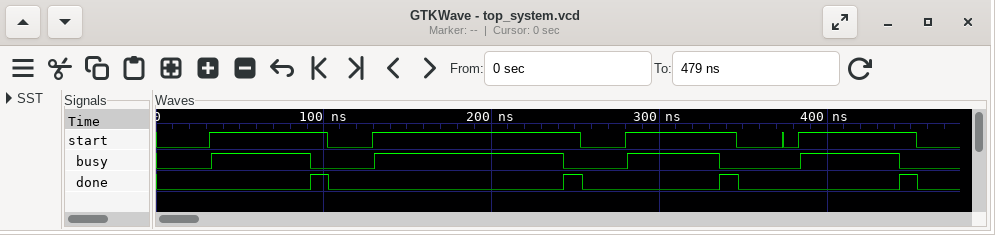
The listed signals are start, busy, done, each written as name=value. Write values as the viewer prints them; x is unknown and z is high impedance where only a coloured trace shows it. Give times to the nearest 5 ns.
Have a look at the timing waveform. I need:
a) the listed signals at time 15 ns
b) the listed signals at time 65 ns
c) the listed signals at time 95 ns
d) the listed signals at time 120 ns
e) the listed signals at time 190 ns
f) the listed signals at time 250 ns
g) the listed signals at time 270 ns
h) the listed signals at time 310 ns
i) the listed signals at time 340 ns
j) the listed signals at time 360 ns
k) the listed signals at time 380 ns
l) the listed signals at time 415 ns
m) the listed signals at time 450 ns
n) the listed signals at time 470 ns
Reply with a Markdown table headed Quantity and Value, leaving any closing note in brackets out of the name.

| Quantity | Value |
|---|---|
| the listed signals at time 15 ns | start=0, busy=0, done=0 |
| the listed signals at time 65 ns | start=1, busy=1, done=0 |
| the listed signals at time 95 ns | start=1, busy=0, done=1 |
| the listed signals at time 120 ns | start=0, busy=0, done=0 |
| the listed signals at time 190 ns | start=1, busy=1, done=0 |
| the listed signals at time 250 ns | start=1, busy=0, done=1 |
| the listed signals at time 270 ns | start=0, busy=0, done=0 |
| the listed signals at time 310 ns | start=1, busy=1, done=0 |
| the listed signals at time 340 ns | start=1, busy=0, done=1 |
| the listed signals at time 360 ns | start=0, busy=0, done=0 |
| the listed signals at time 380 ns | start=0, busy=0, done=0 |
| the listed signals at time 415 ns | start=1, busy=1, done=0 |
| the listed signals at time 450 ns | start=1, busy=0, done=1 |
| the listed signals at time 470 ns | start=0, busy=0, done=0 |
